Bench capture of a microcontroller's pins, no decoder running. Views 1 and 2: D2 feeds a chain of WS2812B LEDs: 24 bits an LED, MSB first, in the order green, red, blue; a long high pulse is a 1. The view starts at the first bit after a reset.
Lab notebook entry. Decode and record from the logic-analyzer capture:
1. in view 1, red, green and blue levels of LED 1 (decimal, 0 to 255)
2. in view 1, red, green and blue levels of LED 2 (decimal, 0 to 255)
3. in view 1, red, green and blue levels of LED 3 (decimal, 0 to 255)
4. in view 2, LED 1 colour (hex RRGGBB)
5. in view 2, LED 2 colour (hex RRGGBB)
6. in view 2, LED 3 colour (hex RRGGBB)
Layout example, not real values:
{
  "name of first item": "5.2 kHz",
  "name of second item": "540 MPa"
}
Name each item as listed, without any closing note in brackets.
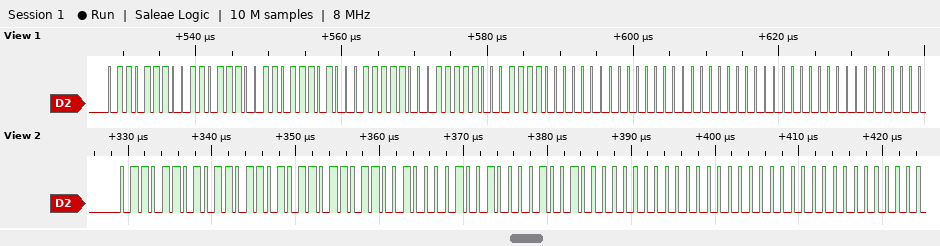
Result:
{
  "in view 1, red, green and blue levels of LED 1": "110, 110, 110",
  "in view 1, red, green and blue levels of LED 2": "143, 143, 143",
  "in view 1, red, green and blue levels of LED 3": "0, 0, 0",
  "in view 2, LED 1 colour": "#6D6D6D",
  "in view 2, LED 2 colour": "#909090",
  "in view 2, LED 3 colour": "#000000"
}
